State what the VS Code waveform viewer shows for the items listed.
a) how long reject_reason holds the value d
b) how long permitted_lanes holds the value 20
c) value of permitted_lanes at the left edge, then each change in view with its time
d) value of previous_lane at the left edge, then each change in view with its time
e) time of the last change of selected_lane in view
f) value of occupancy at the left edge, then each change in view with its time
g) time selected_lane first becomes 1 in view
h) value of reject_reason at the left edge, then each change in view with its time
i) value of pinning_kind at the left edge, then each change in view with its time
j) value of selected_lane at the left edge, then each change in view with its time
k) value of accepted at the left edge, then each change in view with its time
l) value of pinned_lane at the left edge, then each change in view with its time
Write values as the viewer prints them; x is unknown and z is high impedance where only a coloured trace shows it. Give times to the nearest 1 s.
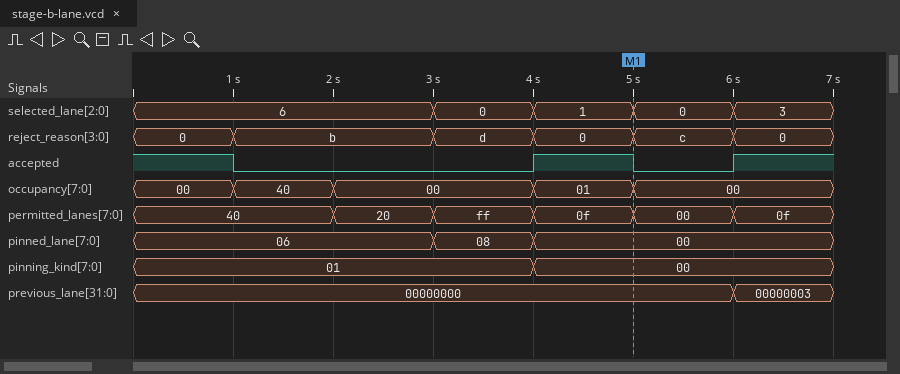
1 s
1 s
40, 20 at 2 s, ff at 3 s, 0f at 4 s, 00 at 5 s, 0f at 6 s
00000000, 00000003 at 6 s
6 s
00, 40 at 1 s, 00 at 2 s, 01 at 4 s, 00 at 5 s
4 s
0, b at 1 s, d at 3 s, 0 at 4 s, c at 5 s, 0 at 6 s
01, 00 at 4 s
6, 0 at 3 s, 1 at 4 s, 0 at 5 s, 3 at 6 s
1, 0 at 1 s, 1 at 4 s, 0 at 5 s, 1 at 6 s
06, 08 at 3 s, 00 at 4 s
